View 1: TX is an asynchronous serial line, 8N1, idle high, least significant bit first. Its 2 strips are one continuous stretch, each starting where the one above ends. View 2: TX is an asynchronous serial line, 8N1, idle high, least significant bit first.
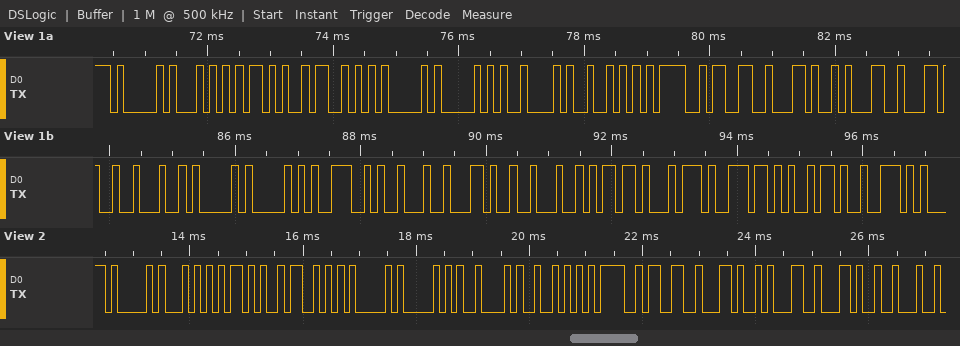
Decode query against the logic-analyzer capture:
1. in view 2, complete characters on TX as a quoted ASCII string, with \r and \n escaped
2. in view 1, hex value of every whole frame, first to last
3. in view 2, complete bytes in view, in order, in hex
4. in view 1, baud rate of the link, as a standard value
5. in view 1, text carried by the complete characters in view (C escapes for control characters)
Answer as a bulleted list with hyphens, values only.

- "AT+SAPBR=3,1,\""
- 41 54 2B 53 41 50 42 52 3D 33 2C 31 2C 22 41 50 4E 22 2C 22 6D 74 6E 69 72
- 41 54 2B 53 41 50 42 52 3D 33 2C 31 2C 22
- 9600 baud
- "AT+SAPBR=3,1,\"APN\",\"mtnir"
